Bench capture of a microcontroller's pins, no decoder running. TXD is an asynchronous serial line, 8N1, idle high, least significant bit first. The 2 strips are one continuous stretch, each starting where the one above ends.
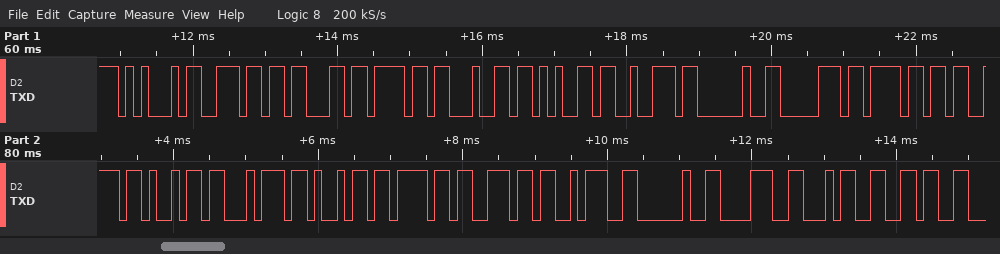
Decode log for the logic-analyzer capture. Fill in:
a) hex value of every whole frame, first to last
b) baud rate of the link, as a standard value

45 6E 63 6F 64 65 72 20 70 6F 73 69 74 69 6F 6E 3A 20 38 34 36
9600 baud
